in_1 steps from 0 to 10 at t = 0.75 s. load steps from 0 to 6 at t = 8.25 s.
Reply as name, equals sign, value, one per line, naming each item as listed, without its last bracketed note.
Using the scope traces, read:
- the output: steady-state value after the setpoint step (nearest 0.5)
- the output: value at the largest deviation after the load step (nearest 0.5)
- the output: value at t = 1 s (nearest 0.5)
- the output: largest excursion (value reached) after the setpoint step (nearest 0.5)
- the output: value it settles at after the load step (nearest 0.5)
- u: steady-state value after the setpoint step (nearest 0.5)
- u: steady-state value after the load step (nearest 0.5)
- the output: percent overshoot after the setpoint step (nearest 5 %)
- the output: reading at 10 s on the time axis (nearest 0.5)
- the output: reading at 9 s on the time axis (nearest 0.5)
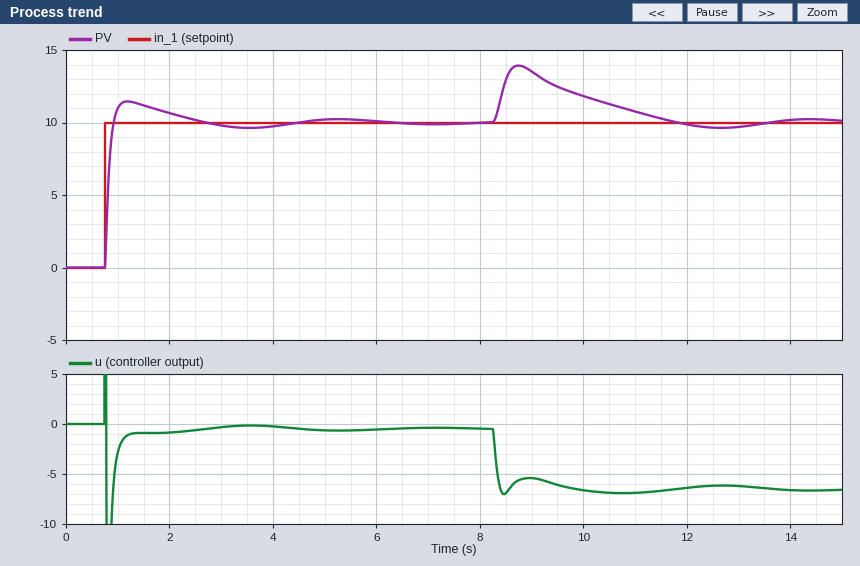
the output: steady-state value after the setpoint step = 10.0
the output: value at the largest deviation after the load step = 14.0
the output: value at t = 1 s = 11.0
the output: largest excursion (value reached) after the setpoint step = 11.5
the output: value it settles at after the load step = 10.0
u: steady-state value after the setpoint step = -0.5
u: steady-state value after the load step = -6.5
the output: percent overshoot after the setpoint step = 15 %
the output: reading at 10 s on the time axis = 12.0
the output: reading at 9 s on the time axis = 13.5
